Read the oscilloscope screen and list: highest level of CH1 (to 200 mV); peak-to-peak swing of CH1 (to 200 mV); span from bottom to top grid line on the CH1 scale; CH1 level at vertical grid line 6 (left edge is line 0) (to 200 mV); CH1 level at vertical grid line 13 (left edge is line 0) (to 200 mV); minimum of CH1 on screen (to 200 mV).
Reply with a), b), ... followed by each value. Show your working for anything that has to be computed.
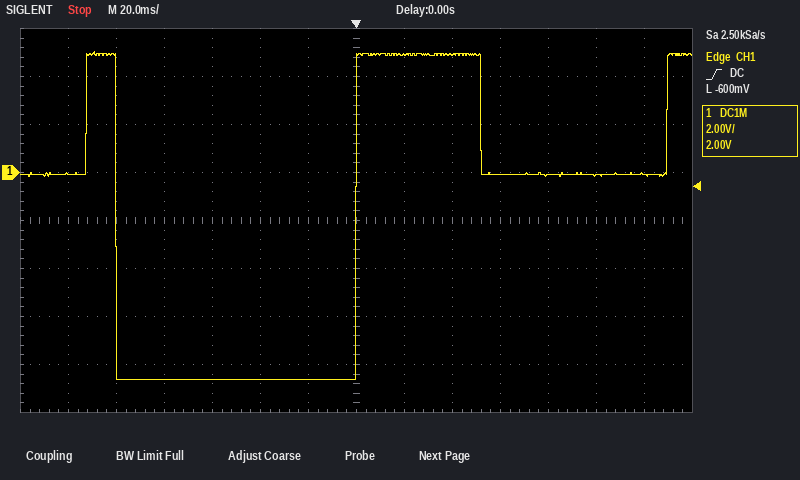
a) 5.0 V
b) 5.0 V − (-8.6 V) = 13.6 V
c) 16 V
d) -8.6 V
e) 0.0 V
f) -8.6 V
